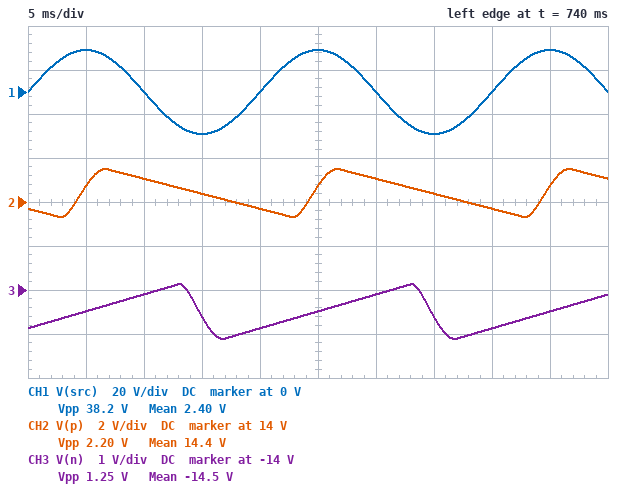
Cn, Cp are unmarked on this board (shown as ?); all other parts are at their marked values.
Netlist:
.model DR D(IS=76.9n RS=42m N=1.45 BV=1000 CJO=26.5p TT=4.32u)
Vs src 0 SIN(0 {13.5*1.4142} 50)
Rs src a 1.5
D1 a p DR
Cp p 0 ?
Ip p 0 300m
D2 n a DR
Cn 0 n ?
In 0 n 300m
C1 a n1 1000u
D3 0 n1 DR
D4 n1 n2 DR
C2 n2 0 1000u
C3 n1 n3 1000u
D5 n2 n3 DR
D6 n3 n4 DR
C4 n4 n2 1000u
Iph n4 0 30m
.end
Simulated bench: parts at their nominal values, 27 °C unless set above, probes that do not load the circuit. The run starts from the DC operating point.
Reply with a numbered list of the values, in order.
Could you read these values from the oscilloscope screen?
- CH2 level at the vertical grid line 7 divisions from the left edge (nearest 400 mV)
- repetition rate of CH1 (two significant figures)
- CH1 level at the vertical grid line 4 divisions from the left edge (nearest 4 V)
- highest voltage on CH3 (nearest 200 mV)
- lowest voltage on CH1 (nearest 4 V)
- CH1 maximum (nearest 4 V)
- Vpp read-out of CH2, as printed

1. 14.4 V
2. 50 Hz
3. 0 V
4. -13.8 V
5. -20 V
6. 20 V
7. 2.20 V
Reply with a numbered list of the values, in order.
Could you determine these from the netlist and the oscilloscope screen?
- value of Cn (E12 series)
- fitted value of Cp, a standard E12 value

1. 3.9 mF
2. 2.2 mF
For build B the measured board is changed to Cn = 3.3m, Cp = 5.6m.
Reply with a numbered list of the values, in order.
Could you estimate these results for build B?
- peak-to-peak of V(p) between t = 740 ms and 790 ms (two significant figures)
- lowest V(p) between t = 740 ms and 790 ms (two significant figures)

1. 880 mV
2. 14 V
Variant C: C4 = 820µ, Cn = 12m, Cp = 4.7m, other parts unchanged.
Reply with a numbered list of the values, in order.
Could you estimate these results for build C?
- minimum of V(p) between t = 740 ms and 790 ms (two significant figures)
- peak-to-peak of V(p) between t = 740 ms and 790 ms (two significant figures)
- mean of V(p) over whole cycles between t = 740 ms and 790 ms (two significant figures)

1. 14 V
2. 1.0 V
3. 15 V
